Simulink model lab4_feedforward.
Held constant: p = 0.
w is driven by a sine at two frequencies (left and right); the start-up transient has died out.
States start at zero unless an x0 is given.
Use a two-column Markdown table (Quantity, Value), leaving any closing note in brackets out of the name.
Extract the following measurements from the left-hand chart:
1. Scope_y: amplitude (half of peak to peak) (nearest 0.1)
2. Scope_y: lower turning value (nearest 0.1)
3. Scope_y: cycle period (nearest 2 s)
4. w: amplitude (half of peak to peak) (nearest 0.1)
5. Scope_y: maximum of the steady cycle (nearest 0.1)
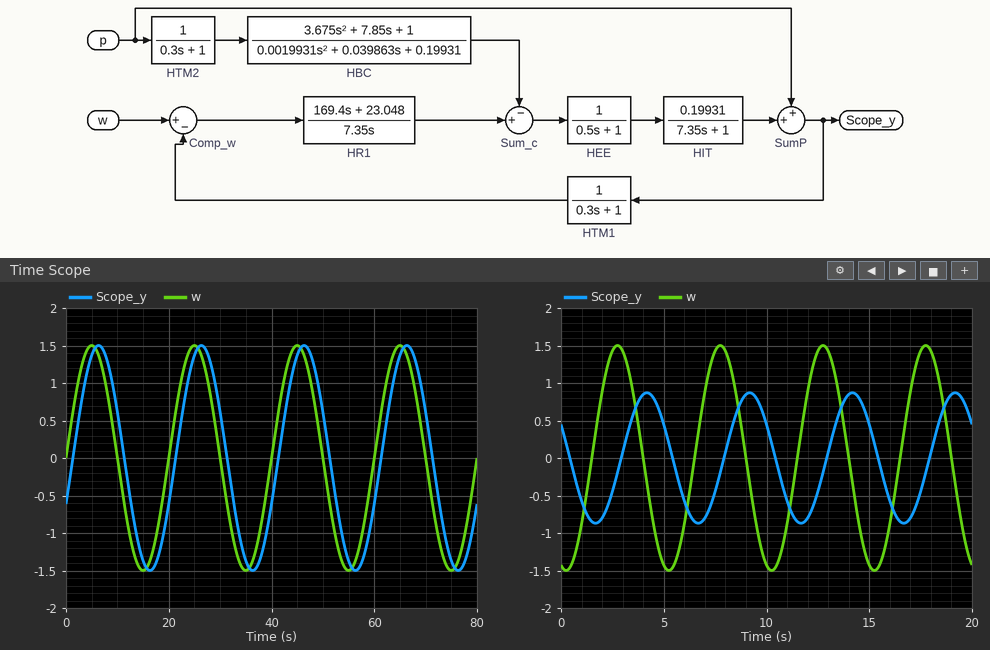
| Quantity | Value |
|---|---|
| Scope_y: amplitude (half of peak to peak) | 1.5 |
| Scope_y: lower turning value | -1.5 |
| Scope_y: cycle period | 20 s |
| w: amplitude (half of peak to peak) | 1.5 |
| Scope_y: maximum of the steady cycle | 1.5 |
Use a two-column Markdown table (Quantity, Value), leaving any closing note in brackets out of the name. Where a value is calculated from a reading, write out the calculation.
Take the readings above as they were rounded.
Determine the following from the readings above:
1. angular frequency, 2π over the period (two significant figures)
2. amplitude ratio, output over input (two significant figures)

| Quantity | Value |
|---|---|
| angular frequency, 2π over the period | 2π / 20 = 0.31 rad/s |
| amplitude ratio, output over input | 1.5 / 1.5 = 1.0 |
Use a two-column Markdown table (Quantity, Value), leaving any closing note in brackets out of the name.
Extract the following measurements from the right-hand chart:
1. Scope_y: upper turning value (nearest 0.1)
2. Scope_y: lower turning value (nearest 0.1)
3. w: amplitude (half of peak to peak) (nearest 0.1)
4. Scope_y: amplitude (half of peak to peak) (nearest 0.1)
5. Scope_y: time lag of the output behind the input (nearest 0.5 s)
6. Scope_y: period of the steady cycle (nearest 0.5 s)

| Quantity | Value |
|---|---|
| Scope_y: upper turning value | 0.9 |
| Scope_y: lower turning value | -0.9 |
| w: amplitude (half of peak to peak) | 1.5 |
| Scope_y: amplitude (half of peak to peak) | 0.9 |
| Scope_y: time lag of the output behind the input | 1.5 s |
| Scope_y: period of the steady cycle | 5.0 s |
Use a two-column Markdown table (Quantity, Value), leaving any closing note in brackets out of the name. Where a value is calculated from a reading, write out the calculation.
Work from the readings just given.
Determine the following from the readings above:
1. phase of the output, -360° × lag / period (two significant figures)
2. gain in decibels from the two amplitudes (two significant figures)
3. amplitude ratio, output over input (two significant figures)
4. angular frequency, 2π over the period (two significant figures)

| Quantity | Value |
|---|---|
| phase of the output, -360° × lag / period | -360 × 1.5 / 5 = -110° |
| gain in decibels from the two amplitudes | 20 log10(0.9 / 1.5) = -4.4 dB |
| amplitude ratio, output over input | 0.9 / 1.5 = 0.60 |
| angular frequency, 2π over the period | 2π / 5 = 1.3 rad/s |
